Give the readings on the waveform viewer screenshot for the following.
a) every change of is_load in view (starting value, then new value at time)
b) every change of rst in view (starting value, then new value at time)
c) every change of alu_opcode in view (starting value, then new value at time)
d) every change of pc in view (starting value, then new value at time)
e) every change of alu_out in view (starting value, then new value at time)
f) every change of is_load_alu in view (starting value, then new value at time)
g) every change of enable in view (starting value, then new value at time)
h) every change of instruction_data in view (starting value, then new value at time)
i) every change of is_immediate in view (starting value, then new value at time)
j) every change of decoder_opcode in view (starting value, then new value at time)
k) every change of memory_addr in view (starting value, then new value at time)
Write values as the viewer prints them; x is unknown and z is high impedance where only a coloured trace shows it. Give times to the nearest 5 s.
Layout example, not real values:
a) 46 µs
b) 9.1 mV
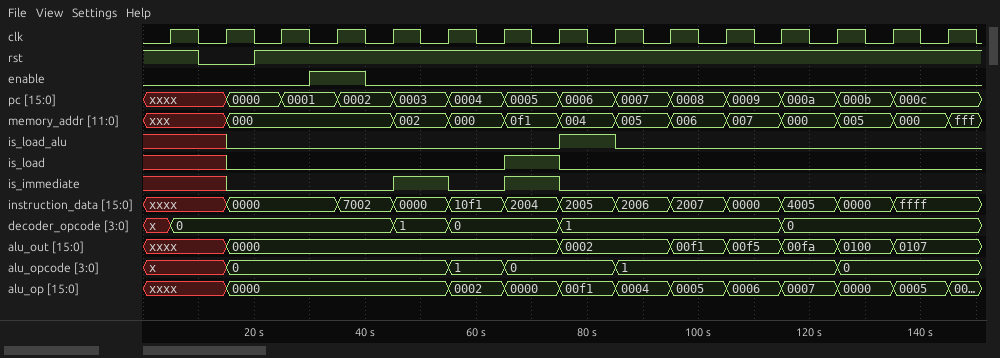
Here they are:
a) x, 0 at 15 s, 1 at 65 s, 0 at 75 s
b) 1, 0 at 10 s, 1 at 20 s
c) x, 0 at 15 s, 1 at 55 s, 0 at 65 s, 1 at 85 s, 0 at 125 s
d) xxxx, 0000 at 15 s, 0001 at 25 s, 0002 at 35 s, 0003 at 45 s, 0004 at 55 s, 0005 at 65 s, 0006 at 75 s, 0007 at 85 s, 0008 at 95 s, 0009 at 105 s, 000a at 115 s, 000b at 125 s, 000c at 135 s
e) xxxx, 0000 at 15 s, 0002 at 75 s, 00f1 at 95 s, 00f5 at 105 s, 00fa at 115 s, 0100 at 125 s, 0107 at 135 s
f) x, 0 at 15 s, 1 at 75 s, 0 at 85 s
g) 0, 1 at 30 s, 0 at 40 s
h) xxxx, 0000 at 15 s, 7002 at 35 s, 0000 at 45 s, 10f1 at 55 s, 2004 at 65 s, 2005 at 75 s, 2006 at 85 s, 2007 at 95 s, 0000 at 105 s, 4005 at 115 s, 0000 at 125 s, ffff at 135 s
i) x, 0 at 15 s, 1 at 45 s, 0 at 55 s, 1 at 65 s, 0 at 75 s
j) x, 0 at 5 s, 1 at 45 s, 0 at 55 s, 1 at 75 s, 0 at 115 s
k) xxx, 000 at 15 s, 002 at 45 s, 000 at 55 s, 0f1 at 65 s, 004 at 75 s, 005 at 85 s, 006 at 95 s, 007 at 105 s, 000 at 115 s, 005 at 125 s, 000 at 135 s, fff at 145 s
